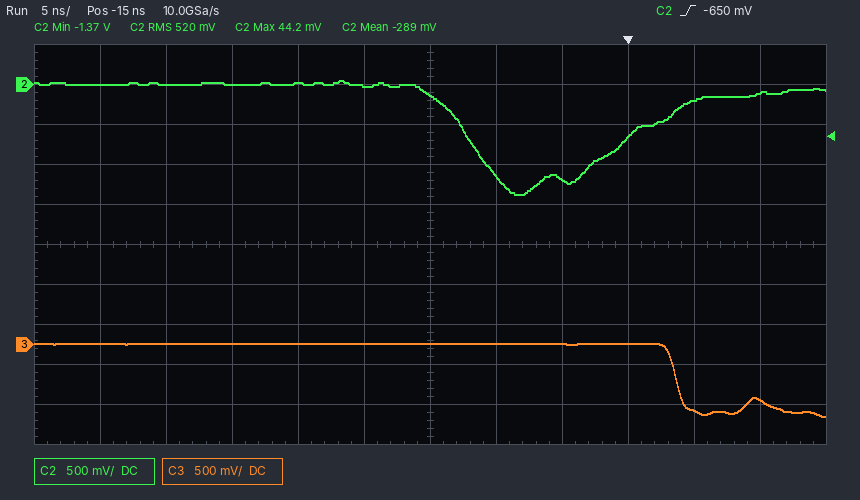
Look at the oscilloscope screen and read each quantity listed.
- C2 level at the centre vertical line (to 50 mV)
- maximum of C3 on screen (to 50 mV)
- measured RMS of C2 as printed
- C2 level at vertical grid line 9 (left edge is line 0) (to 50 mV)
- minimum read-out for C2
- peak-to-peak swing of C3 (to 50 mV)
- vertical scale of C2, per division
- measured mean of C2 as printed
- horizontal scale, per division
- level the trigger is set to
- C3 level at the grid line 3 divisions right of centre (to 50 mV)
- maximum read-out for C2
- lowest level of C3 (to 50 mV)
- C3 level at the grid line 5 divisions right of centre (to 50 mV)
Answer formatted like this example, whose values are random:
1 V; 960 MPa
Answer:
-150 mV; 0 mV; 520 mV; -650 mV; -1.37 V; 900 mV; 500 mV; -289 mV; 5 ns; -650 mV; 0 mV; 44.2 mV; -900 mV; -700 mV
